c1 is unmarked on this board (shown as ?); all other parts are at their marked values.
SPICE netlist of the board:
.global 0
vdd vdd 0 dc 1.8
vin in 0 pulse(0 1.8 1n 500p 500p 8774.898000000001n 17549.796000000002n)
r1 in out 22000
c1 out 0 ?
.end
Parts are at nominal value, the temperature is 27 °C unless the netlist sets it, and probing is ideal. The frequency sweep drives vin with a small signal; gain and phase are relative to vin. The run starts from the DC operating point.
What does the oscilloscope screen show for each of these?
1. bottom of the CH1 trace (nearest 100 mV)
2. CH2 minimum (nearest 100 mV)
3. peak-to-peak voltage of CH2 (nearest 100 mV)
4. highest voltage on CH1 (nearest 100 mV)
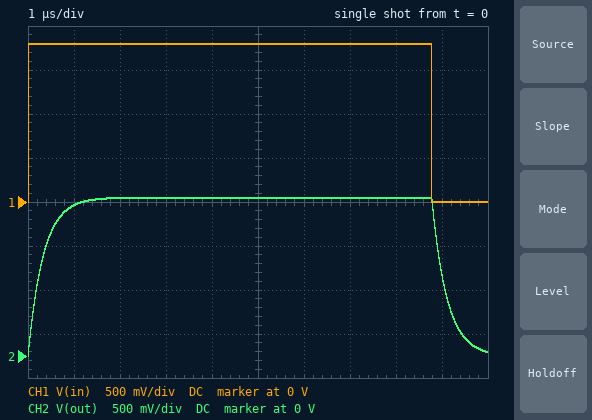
0 V
0 V
1.8 V
1.8 V
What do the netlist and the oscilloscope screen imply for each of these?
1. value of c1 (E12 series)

15 pF
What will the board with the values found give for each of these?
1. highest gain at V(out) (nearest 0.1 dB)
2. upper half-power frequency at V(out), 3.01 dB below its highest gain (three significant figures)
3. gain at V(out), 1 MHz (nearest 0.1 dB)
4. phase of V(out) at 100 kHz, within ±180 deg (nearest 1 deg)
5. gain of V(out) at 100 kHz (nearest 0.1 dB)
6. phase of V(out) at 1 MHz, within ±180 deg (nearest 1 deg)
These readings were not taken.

0 dB
482 kHz
-7.2 dB
-12 deg
-0.2 dB
-64 deg
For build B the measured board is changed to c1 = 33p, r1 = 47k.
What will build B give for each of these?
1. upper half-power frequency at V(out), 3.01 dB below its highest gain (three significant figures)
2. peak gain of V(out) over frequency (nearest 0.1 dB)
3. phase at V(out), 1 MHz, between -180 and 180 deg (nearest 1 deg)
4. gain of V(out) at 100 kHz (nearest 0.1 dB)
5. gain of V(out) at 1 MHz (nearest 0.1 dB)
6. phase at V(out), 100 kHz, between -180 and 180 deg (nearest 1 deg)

103 kHz
0 dB
-84 deg
-2.9 dB
-19.8 dB
-44 deg
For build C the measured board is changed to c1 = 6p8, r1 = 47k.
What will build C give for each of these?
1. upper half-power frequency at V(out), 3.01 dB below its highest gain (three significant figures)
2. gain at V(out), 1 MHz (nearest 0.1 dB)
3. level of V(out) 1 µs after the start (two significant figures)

498 kHz
-7.0 dB
1.7 V
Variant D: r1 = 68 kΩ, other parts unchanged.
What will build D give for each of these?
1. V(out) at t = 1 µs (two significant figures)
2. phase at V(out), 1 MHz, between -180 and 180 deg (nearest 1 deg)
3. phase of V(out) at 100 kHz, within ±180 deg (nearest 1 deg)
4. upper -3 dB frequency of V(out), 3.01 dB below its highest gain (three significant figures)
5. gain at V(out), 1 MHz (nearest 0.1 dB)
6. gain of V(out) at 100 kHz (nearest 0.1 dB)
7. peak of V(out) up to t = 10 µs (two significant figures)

1.1 V
-81 deg
-33 deg
156 kHz
-16.2 dB
-1.5 dB
1.8 V
